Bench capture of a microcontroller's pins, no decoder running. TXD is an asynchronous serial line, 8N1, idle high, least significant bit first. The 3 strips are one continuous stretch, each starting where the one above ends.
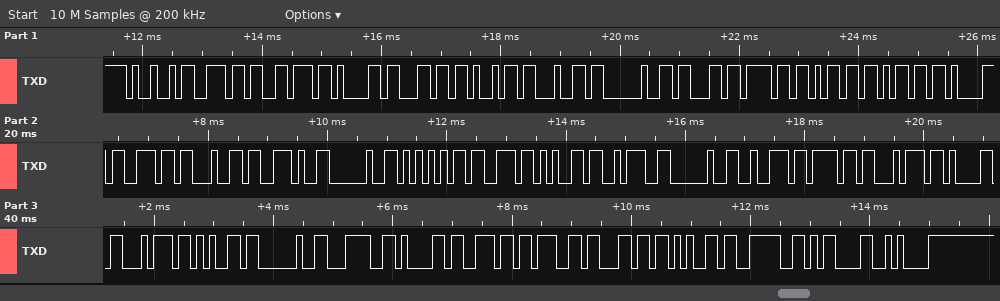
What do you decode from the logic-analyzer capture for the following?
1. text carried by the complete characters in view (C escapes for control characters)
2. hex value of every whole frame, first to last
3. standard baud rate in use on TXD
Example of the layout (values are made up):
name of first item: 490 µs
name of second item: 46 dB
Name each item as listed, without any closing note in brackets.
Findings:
text carried by the complete characters in view: "Invalid command. Use: rotate <angle>\r\n"
hex value of every whole frame, first to last: 49 6E 76 61 6C 69 64 20 63 6F 6D 6D 61 6E 64 2E 20 55 73 65 3A 20 72 6F 74 61 74 65 20 3C 61 6E 67 6C 65 3E 0D 0A
standard baud rate in use on TXD: 9600 baud
